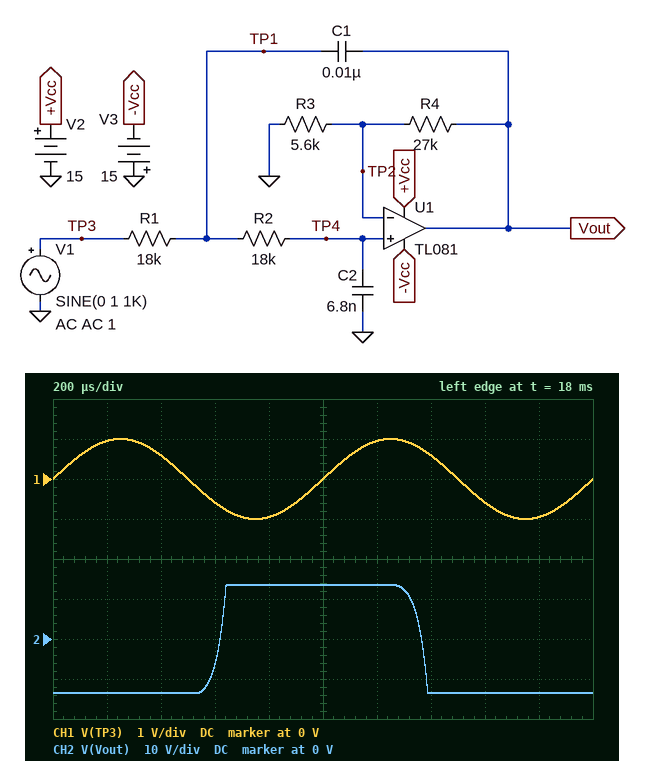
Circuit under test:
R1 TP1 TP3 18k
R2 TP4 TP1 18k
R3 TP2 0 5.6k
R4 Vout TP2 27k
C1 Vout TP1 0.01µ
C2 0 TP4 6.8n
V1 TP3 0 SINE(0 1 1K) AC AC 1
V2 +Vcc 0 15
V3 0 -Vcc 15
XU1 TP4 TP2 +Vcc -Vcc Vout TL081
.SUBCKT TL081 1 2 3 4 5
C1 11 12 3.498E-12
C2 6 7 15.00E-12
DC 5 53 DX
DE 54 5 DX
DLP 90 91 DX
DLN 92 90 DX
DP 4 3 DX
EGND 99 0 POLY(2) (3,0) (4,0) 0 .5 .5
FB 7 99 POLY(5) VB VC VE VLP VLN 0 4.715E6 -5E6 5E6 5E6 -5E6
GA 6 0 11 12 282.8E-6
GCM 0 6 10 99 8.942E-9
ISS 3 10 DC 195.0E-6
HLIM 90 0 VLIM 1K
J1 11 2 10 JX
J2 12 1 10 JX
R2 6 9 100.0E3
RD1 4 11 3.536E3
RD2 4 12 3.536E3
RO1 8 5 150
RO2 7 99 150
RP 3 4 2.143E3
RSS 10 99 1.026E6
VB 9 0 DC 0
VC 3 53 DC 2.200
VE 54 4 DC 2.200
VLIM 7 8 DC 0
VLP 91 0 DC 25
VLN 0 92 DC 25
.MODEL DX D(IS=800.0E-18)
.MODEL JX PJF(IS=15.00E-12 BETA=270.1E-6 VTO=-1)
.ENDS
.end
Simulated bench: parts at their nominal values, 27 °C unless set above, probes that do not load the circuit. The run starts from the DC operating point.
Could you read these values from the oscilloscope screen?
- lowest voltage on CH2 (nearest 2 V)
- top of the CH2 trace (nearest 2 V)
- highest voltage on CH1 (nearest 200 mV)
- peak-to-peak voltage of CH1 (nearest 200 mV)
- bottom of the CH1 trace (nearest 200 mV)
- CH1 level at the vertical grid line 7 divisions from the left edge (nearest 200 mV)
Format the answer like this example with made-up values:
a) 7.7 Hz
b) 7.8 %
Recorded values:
a) -14 V
b) 14 V
c) 1.0 V
d) 2.0 V
e) -1.0 V
f) 600 mV
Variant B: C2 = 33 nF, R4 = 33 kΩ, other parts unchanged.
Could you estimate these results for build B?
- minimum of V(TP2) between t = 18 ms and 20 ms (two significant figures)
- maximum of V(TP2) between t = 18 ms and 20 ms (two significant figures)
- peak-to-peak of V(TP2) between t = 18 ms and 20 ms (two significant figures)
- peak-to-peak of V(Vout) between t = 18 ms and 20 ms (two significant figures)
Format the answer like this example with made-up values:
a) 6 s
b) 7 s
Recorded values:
a) -300 mV
b) 300 mV
c) 600 mV
d) 4.1 V
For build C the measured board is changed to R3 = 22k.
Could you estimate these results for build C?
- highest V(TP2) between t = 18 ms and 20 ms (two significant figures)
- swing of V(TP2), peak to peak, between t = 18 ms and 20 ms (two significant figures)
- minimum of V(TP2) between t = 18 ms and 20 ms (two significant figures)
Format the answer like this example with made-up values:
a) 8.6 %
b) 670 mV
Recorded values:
a) 5.1 V
b) 10 V
c) -5.1 V
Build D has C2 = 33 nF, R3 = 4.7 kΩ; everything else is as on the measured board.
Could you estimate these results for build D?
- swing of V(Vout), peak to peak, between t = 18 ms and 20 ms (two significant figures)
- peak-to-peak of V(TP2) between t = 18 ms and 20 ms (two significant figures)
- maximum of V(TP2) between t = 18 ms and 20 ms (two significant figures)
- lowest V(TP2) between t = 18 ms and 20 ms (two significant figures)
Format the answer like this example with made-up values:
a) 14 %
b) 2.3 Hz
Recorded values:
a) 4.0 V
b) 590 mV
c) 300 mV
d) -300 mV
